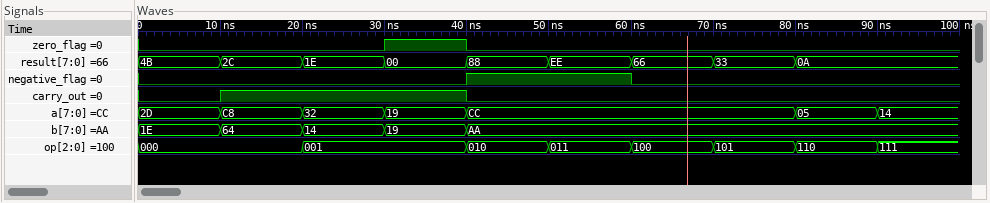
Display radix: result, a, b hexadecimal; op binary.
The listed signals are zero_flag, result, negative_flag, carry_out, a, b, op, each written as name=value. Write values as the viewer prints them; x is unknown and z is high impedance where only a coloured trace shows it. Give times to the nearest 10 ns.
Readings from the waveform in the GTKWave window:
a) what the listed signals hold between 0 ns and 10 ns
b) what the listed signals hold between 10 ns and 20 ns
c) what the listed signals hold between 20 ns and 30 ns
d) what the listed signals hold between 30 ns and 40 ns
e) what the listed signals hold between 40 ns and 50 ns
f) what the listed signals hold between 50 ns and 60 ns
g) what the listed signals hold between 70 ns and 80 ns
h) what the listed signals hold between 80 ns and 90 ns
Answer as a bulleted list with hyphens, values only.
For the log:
- zero_flag=0, result=4B, negative_flag=0, carry_out=0, a=2D, b=1E, op=000
- zero_flag=0, result=2C, negative_flag=0, carry_out=1, a=C8, b=64, op=000
- zero_flag=0, result=1E, negative_flag=0, carry_out=1, a=32, b=14, op=001
- zero_flag=1, result=00, negative_flag=0, carry_out=1, a=19, b=19, op=001
- zero_flag=0, result=88, negative_flag=1, carry_out=0, a=CC, b=AA, op=010
- zero_flag=0, result=EE, negative_flag=1, carry_out=0, a=CC, b=AA, op=011
- zero_flag=0, result=33, negative_flag=0, carry_out=0, a=CC, b=AA, op=101
- zero_flag=0, result=0A, negative_flag=0, carry_out=0, a=05, b=AA, op=110
